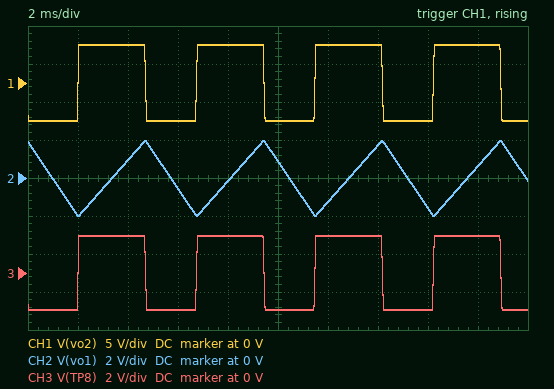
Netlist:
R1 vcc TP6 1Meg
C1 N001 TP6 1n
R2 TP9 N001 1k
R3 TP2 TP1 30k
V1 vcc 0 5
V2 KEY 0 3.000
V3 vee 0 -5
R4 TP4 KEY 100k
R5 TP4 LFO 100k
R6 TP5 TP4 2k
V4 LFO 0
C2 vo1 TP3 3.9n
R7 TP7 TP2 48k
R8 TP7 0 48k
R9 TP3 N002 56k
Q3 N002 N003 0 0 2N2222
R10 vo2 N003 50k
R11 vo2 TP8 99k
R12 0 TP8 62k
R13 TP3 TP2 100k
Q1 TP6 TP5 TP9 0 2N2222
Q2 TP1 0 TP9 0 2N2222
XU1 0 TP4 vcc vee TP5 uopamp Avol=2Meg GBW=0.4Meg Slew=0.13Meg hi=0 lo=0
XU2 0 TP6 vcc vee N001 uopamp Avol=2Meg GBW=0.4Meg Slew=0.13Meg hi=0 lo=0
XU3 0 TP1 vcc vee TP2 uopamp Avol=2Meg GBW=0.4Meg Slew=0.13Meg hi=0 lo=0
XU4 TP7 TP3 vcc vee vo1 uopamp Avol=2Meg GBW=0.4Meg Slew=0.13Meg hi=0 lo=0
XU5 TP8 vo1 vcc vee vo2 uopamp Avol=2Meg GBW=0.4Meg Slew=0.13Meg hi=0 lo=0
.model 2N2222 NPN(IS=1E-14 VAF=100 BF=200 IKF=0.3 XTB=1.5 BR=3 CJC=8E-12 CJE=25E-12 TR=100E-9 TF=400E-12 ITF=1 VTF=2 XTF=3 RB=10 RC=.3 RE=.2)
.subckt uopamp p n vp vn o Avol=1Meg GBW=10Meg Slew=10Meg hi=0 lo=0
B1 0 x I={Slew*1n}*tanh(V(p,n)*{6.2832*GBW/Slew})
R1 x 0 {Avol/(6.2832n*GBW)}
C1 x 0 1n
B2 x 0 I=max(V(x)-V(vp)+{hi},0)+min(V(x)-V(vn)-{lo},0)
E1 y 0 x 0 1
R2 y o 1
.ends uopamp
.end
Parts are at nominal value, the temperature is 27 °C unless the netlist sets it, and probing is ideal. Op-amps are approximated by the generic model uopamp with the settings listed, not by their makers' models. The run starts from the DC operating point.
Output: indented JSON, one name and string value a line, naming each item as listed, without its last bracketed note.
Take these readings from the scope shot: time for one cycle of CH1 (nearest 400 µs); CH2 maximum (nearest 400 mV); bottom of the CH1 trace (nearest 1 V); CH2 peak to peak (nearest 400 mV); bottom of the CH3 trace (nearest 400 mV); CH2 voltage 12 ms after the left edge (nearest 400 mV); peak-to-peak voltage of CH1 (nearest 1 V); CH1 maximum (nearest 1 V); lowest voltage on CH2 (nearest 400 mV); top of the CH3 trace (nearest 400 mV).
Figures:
{
  "time for one cycle of CH1": "4.8 ms",
  "CH2 maximum": "2.0 V",
  "bottom of the CH1 trace": "-5 V",
  "CH2 peak to peak": "4.0 V",
  "bottom of the CH3 trace": "-2.0 V",
  "CH2 voltage 12 ms after the left edge": "-1.2 V",
  "peak-to-peak voltage of CH1": "10 V",
  "CH1 maximum": "5 V",
  "lowest voltage on CH2": "-2.0 V",
  "top of the CH3 trace": "2.0 V"
}
